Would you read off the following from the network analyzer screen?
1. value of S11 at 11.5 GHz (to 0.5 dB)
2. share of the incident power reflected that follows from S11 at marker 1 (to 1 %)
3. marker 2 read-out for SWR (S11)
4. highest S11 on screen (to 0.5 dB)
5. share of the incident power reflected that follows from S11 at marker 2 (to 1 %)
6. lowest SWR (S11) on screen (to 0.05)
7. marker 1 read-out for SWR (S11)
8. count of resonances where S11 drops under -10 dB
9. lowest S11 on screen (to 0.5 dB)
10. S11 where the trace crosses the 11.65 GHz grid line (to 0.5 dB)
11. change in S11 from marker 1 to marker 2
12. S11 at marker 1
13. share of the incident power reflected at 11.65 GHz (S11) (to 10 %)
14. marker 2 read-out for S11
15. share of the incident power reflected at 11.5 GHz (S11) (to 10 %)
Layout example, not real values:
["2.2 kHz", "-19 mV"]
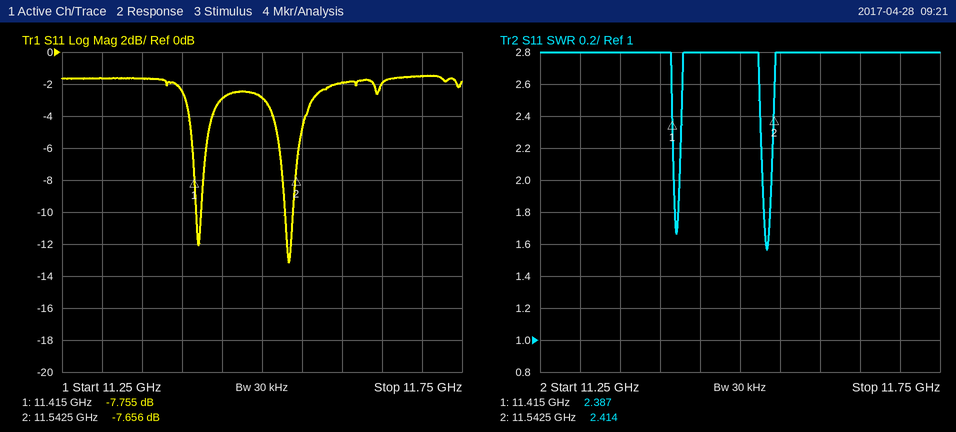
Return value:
["-3.0 dB", "17 %", "2.414", "-1.5 dB", "17 %", "1.55", "2.387", "2", "-13.0 dB", "-2.0 dB", "0.099 dB", "-7.755 dB", "60 %", "-7.656 dB", "50 %"]
